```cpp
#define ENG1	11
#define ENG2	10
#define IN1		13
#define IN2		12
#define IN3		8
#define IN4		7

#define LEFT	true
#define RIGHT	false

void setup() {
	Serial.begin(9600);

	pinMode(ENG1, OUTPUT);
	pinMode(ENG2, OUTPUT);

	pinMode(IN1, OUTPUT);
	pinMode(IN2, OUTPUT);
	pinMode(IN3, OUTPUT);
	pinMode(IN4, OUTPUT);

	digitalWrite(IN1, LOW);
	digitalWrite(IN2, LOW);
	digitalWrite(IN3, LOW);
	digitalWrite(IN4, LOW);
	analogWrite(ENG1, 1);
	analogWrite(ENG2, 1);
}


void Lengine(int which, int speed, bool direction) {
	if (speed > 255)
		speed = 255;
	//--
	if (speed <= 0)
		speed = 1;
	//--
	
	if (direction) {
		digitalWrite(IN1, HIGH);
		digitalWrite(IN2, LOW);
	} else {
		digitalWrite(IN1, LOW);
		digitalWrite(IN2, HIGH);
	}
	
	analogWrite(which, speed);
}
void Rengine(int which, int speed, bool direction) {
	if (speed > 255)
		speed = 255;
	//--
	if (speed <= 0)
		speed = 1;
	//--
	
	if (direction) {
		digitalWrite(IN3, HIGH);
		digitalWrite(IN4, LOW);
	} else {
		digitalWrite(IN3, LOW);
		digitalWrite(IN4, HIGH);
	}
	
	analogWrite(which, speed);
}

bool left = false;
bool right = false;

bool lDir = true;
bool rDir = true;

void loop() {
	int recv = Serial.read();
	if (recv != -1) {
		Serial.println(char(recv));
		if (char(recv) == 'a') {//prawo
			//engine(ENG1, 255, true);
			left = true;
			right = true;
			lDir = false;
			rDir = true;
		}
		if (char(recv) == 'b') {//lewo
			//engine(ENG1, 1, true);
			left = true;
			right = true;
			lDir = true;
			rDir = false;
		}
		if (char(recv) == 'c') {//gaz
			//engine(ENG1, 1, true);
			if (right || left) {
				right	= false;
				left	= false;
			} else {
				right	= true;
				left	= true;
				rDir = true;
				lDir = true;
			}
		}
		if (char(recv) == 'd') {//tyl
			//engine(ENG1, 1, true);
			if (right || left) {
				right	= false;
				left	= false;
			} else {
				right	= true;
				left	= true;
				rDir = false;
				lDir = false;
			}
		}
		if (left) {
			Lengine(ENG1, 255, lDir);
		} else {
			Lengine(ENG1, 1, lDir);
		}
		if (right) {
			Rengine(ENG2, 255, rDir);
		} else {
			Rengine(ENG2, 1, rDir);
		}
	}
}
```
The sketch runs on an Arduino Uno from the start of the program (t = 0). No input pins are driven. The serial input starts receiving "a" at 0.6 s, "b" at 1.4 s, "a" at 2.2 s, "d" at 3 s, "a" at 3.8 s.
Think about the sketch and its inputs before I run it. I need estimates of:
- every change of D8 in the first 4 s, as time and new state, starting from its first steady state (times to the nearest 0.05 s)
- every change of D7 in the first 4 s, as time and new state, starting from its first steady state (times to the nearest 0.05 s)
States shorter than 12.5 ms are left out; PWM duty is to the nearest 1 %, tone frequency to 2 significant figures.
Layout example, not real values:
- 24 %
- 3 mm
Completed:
- 0 s low; 0.6 s high; 1.4 s low; 2.2 s high
- 0 s low; 1.4 s high; 2.2 s low
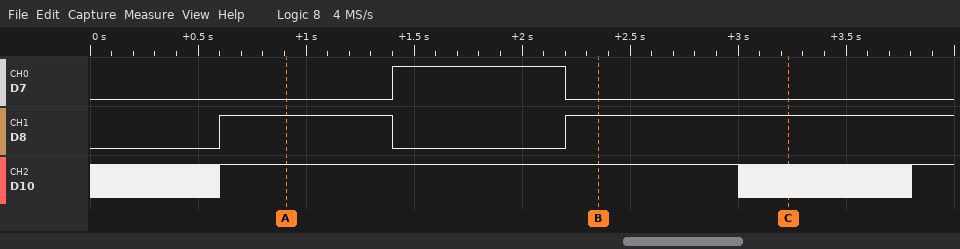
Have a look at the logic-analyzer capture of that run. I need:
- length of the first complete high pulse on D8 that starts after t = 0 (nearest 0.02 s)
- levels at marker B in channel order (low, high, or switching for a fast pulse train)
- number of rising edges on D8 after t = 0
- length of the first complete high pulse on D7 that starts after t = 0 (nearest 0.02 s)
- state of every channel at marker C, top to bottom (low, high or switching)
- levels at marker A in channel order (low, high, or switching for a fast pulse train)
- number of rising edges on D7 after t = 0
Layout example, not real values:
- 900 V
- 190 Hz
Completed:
- 0.80 s
- D7 low, D8 high, D10 high
- 2
- 0.80 s
- D7 low, D8 high, D10 switching
- D7 low, D8 high, D10 high
- 1
